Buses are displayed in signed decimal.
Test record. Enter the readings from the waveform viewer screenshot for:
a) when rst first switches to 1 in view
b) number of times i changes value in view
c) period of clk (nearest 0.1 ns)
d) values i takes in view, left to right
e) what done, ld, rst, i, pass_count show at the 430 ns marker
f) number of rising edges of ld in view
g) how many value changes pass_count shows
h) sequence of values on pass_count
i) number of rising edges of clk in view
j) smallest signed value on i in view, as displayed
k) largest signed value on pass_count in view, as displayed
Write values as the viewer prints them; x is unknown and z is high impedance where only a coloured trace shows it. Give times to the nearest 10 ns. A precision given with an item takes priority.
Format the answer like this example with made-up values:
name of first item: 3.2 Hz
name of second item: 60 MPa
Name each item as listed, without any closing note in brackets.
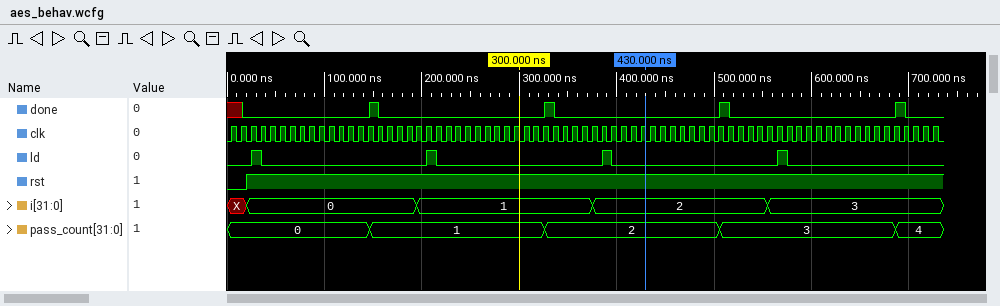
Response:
when rst first switches to 1 in view: 20 ns
number of times i changes value in view: 4
period of clk: 10 ns
values i takes in view, left to right: X, 0, 1, 2, 3
what done, ld, rst, i, pass_count show at the 430 ns marker: done=0, ld=0, rst=1, i=2, pass_count=2
number of rising edges of ld in view: 4
how many value changes pass_count shows: 4
sequence of values on pass_count: 0, 1, 2, 3, 4
number of rising edges of clk in view: 73
smallest signed value on i in view, as displayed: 0
largest signed value on pass_count in view, as displayed: 4
